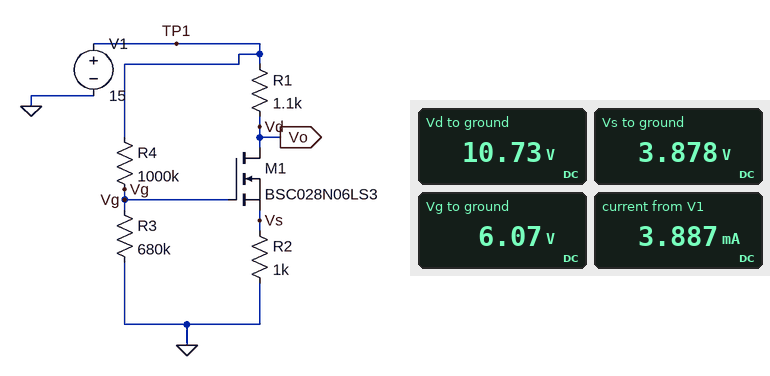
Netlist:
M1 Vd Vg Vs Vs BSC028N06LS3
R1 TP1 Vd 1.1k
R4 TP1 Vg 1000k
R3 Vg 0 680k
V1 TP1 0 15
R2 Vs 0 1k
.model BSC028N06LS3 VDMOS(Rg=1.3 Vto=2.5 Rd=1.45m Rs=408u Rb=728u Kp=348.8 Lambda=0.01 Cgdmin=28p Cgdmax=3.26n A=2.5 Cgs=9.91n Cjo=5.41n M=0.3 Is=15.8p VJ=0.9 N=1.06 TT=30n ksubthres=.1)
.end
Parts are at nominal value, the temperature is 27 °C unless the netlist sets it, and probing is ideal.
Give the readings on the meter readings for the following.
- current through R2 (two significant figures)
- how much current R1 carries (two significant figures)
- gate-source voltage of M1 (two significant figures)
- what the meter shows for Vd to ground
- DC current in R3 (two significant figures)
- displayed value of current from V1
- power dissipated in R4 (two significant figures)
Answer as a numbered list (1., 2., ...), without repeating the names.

1. 3.9 mA
2. 3.9 mA
3. 2.2 V
4. 10.73 V
5. 8.9 µA
6. 3.887 mA
7. 80 µW
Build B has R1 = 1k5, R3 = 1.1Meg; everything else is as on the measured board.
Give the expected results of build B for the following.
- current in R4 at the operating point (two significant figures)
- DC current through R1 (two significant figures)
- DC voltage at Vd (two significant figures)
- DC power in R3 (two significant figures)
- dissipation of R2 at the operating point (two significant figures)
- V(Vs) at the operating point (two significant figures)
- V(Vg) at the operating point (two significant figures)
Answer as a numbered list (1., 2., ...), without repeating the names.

1. 7.1 µA
2. 5.6 mA
3. 6.5 V
4. 56 µW
5. 32 mW
6. 5.6 V
7. 7.9 V
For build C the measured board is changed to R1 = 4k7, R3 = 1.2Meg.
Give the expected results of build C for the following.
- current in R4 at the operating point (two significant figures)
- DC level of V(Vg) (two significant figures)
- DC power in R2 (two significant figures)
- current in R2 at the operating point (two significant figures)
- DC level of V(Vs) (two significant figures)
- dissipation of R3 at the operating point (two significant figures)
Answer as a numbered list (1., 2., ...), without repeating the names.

1. 6.8 µA
2. 8.2 V
3. 6.9 mW
4. 2.6 mA
5. 2.6 V
6. 56 µW
